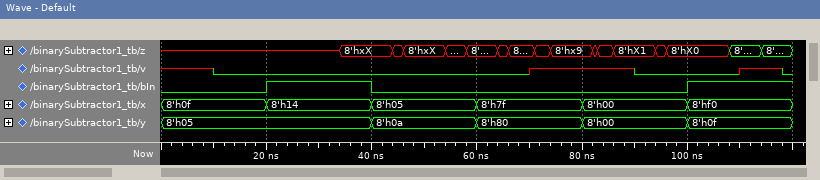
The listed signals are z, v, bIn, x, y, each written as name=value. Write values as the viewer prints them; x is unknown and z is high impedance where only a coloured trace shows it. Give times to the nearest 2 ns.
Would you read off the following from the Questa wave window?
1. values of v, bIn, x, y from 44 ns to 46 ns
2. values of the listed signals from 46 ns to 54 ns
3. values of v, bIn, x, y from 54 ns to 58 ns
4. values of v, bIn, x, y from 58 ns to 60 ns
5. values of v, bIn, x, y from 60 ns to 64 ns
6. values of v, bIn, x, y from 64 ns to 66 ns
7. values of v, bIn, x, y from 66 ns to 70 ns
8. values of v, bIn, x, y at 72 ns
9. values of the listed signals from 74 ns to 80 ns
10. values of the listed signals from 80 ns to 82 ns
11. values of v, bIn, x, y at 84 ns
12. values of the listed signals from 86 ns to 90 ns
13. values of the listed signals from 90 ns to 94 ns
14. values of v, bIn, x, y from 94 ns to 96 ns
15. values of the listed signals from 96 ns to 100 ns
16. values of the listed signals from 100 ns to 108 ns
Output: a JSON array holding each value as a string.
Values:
["v=0, bIn=0, x=8'h05, y=8'h0a", "z=8'hxX, v=0, bIn=0, x=8'h05, y=8'h0a", "v=0, bIn=0, x=8'h05, y=8'h0a", "v=0, bIn=0, x=8'h05, y=8'h0a", "v=0, bIn=0, x=8'h7f, y=8'h80", "v=0, bIn=0, x=8'h7f, y=8'h80", "v=0, bIn=0, x=8'h7f, y=8'h80", "v=x, bIn=0, x=8'h7f, y=8'h80", "z=8'hx9, v=x, bIn=0, x=8'h7f, y=8'h80", "z=8'hx9, v=x, bIn=0, x=8'h00, y=8'h00", "v=x, bIn=0, x=8'h00, y=8'h00", "z=8'hX1, v=x, bIn=0, x=8'h00, y=8'h00", "z=8'hX1, v=0, bIn=0, x=8'h00, y=8'h00", "v=0, bIn=0, x=8'h00, y=8'h00", "z=8'hX0, v=0, bIn=0, x=8'h00, y=8'h00", "z=8'hX0, v=0, bIn=1, x=8'hf0, y=8'h0f"]
